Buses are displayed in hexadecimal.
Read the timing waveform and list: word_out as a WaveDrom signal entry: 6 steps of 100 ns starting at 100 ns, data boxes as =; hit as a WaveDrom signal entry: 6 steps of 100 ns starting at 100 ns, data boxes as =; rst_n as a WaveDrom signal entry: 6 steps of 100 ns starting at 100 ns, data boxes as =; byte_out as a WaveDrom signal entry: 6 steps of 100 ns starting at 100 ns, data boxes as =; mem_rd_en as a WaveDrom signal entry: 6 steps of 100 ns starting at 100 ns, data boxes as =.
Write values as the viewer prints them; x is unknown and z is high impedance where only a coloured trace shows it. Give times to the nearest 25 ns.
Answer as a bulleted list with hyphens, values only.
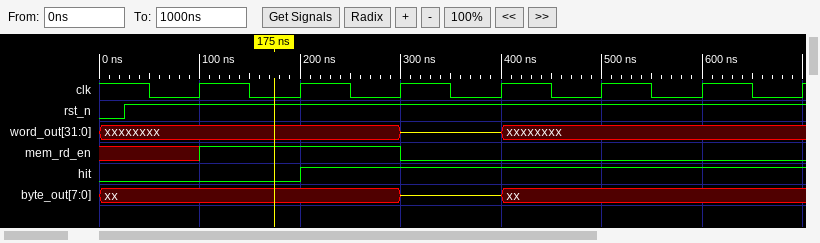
- {name: 'word_out', wave: 'x.zx..'}
- {name: 'hit', wave: '01....'}
- {name: 'rst_n', wave: '1.....'}
- {name: 'byte_out', wave: 'x.zx..'}
- {name: 'mem_rd_en', wave: '1.0...'}
